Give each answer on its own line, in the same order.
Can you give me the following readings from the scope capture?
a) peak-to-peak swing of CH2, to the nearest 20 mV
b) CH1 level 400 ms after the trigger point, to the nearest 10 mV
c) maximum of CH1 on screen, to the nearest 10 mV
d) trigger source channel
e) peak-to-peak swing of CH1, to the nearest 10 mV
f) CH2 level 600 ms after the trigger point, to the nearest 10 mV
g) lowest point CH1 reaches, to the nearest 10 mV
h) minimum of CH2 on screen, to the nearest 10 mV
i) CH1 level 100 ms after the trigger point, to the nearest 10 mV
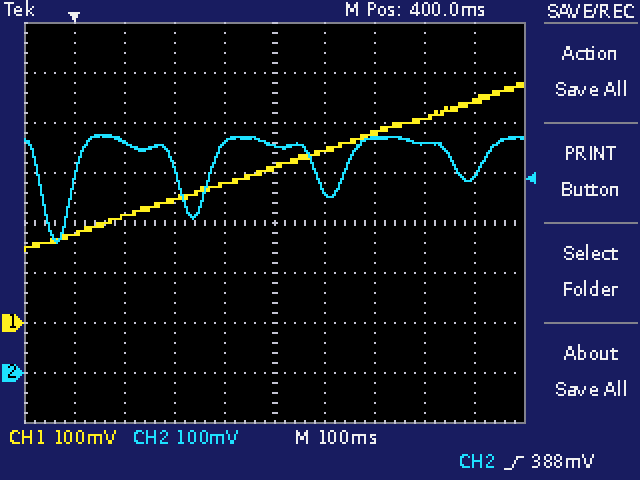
220 mV
310 mV
480 mV
CH2
340 mV
470 mV
140 mV
260 mV
210 mV
